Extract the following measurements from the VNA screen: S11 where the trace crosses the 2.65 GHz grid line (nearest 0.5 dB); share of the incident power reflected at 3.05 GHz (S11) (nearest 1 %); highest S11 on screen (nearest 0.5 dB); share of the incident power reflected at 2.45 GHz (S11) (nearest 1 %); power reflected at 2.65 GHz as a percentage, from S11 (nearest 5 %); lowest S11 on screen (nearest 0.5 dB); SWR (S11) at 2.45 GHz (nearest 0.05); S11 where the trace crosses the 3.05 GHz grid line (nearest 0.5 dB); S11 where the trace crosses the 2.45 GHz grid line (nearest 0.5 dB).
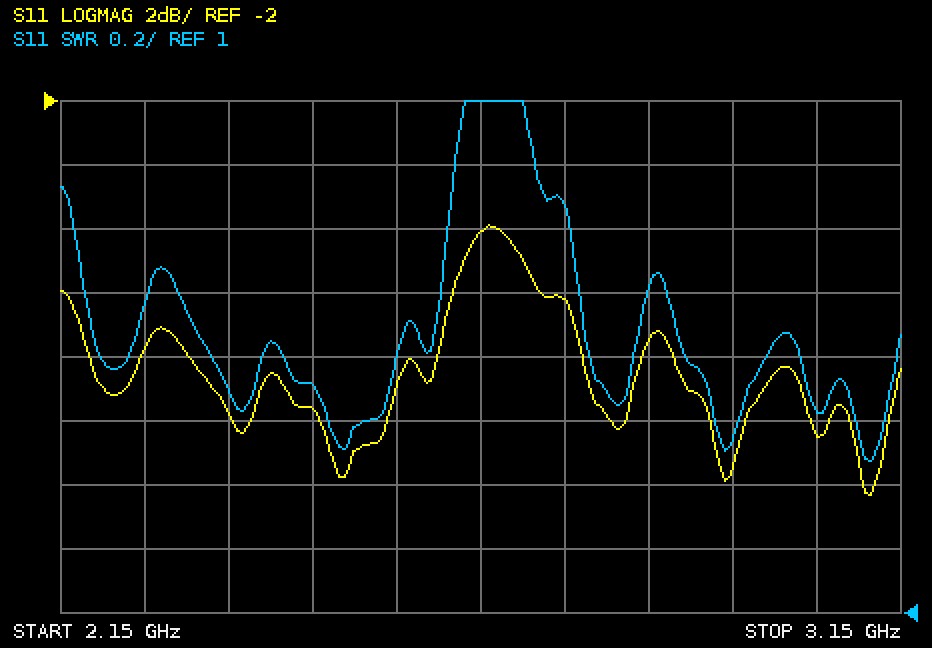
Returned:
-6.0 dB
6 %
-6.0 dB
7 %
25 %
-14.5 dB
1.70
-12.5 dB
-11.5 dB
